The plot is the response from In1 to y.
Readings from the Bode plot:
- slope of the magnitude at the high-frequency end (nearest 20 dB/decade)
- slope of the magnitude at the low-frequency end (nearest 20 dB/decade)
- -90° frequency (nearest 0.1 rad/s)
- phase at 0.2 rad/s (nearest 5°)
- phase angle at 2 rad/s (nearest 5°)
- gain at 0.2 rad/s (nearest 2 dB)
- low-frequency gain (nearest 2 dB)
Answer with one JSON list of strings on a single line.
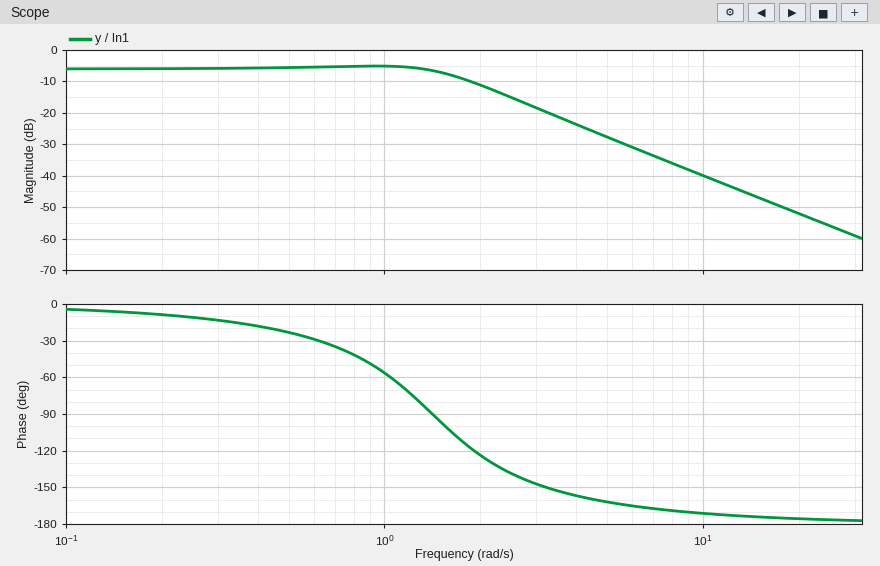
["-40 dB/decade", "0 dB/decade", "1.4 rad/s", "-10°", "-125°", "-6 dB", "-6 dB"]
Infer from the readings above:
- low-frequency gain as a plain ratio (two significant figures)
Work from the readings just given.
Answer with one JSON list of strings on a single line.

["0.50"]
